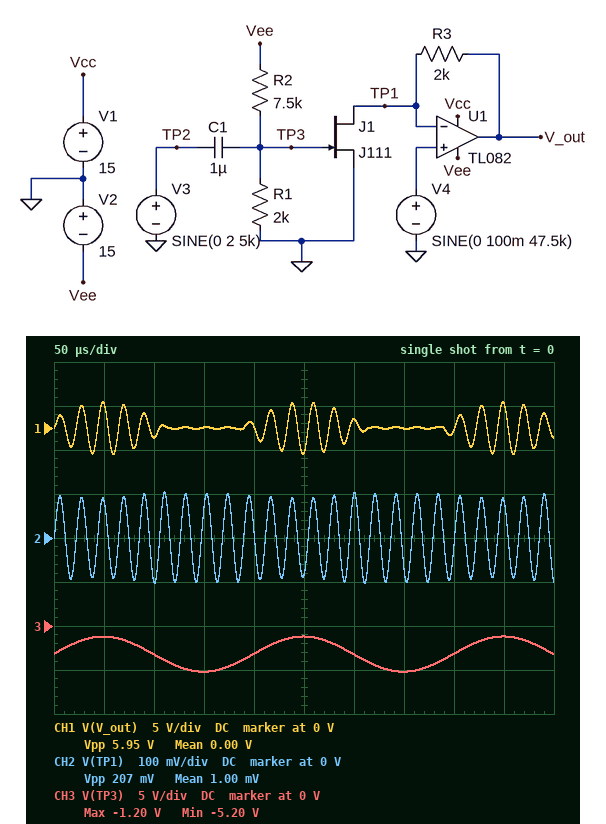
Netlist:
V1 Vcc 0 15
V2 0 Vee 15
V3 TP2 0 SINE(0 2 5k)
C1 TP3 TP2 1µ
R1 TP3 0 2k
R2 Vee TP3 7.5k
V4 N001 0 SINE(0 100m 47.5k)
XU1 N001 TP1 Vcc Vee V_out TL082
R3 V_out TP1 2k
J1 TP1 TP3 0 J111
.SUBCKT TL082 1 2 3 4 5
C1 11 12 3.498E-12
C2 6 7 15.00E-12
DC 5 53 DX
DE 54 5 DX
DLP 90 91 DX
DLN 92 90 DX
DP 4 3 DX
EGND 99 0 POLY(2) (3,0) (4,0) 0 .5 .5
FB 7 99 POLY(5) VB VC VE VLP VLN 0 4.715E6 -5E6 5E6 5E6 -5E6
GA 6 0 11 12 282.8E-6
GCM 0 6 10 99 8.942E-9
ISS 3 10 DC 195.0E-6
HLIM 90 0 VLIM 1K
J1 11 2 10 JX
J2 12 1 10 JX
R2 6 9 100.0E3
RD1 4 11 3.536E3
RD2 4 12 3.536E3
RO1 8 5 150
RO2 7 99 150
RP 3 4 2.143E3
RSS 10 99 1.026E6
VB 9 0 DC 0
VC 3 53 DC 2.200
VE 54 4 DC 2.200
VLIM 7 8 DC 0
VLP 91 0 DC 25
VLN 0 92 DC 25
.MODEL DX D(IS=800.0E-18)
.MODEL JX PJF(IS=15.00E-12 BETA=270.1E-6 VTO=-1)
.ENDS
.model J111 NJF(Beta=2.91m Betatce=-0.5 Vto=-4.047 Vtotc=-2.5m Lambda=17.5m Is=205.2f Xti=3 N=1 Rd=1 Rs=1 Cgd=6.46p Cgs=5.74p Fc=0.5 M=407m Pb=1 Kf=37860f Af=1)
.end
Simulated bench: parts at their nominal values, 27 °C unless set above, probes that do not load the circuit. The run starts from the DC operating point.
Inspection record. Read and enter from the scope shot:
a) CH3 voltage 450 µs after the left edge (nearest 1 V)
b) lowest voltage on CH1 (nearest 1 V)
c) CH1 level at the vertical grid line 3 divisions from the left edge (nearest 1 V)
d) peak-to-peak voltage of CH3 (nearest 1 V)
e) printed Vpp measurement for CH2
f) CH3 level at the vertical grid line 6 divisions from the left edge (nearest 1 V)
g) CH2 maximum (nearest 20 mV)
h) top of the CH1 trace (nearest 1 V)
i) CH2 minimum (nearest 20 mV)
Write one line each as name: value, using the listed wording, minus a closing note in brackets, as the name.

CH3 voltage 450 µs after the left edge: -1 V
lowest voltage on CH1: -3 V
CH1 level at the vertical grid line 3 divisions from the left edge: 0 V
peak-to-peak voltage of CH3: 4 V
printed Vpp measurement for CH2: 207 mV
CH3 level at the vertical grid line 6 divisions from the left edge: -3 V
CH2 maximum: 100 mV
top of the CH1 trace: 3 V
CH2 minimum: -100 mV
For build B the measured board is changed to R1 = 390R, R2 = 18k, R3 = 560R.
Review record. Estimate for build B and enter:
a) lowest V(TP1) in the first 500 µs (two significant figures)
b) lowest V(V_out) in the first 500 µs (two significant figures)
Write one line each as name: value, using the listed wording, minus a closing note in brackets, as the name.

lowest V(TP1) in the first 500 µs: -110 mV
lowest V(V_out) in the first 500 µs: -13 V
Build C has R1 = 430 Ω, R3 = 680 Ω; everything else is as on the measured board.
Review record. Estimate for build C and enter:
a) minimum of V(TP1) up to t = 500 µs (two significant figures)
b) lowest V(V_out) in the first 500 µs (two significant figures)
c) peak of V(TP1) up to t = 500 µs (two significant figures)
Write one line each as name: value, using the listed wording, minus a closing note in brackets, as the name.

minimum of V(TP1) up to t = 500 µs: -110 mV
lowest V(V_out) in the first 500 µs: -13 V
peak of V(TP1) up to t = 500 µs: 110 mV
